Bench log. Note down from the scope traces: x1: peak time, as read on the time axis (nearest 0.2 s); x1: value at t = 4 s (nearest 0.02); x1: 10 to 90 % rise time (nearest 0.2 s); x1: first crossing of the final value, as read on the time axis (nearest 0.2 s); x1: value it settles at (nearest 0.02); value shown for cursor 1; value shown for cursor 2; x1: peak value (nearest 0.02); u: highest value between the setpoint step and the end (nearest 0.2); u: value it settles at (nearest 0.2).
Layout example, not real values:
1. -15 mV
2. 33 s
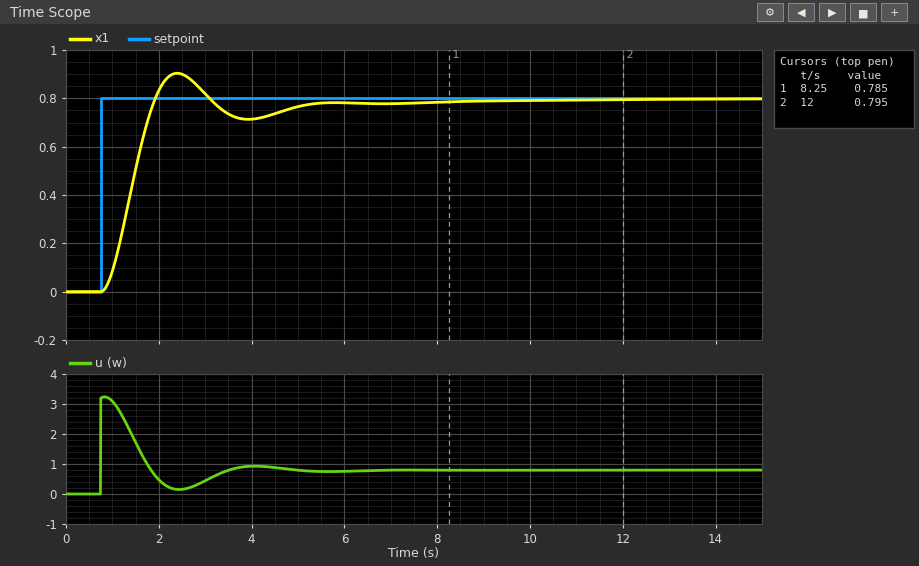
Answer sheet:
1. 2.4 s
2. 0.72
3. 0.8 s
4. 2.0 s
5. 0.80
6. 0.785
7. 0.795
8. 0.90
9. 3.2
10. 0.8
